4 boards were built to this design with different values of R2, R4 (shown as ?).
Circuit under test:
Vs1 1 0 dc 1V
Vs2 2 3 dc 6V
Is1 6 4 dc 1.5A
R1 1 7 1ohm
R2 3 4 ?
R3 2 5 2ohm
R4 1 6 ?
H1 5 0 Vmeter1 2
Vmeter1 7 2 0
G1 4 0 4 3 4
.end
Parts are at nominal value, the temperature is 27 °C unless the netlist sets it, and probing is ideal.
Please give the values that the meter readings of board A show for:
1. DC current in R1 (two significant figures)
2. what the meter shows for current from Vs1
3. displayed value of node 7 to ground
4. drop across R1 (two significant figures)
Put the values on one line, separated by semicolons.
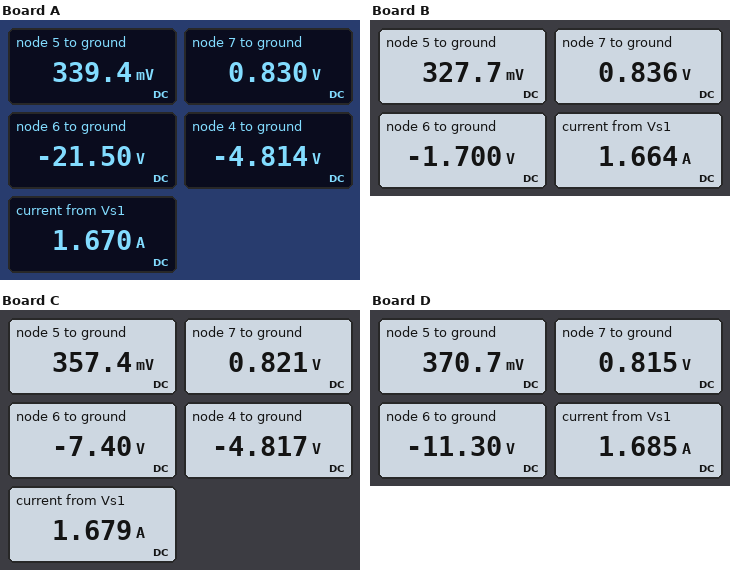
170 mA; 1.670 A; 0.830 V; 170 mV
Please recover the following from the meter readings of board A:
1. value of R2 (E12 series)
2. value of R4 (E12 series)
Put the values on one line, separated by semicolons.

4.7 Ω; 15 Ω
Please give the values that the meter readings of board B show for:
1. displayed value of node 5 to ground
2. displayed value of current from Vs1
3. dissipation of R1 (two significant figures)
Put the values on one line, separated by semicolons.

327.7 mV; 1.664 A; 27 mW
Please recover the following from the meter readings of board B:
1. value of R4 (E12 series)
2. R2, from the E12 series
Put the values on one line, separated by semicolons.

1.8 Ω; 3.9 Ω
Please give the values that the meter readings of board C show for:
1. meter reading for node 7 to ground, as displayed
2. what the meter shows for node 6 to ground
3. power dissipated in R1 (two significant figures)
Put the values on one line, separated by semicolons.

0.821 V; -7.40 V; 32 mW
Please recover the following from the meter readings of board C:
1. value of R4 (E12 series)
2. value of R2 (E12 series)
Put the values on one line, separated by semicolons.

5.6 Ω; 6.8 Ω
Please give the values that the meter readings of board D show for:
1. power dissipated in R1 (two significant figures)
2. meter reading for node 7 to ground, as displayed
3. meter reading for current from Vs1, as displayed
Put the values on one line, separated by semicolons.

34 mW; 0.815 V; 1.685 A
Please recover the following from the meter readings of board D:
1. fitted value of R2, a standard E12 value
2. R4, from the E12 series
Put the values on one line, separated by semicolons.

10 Ω; 8.2 Ω
